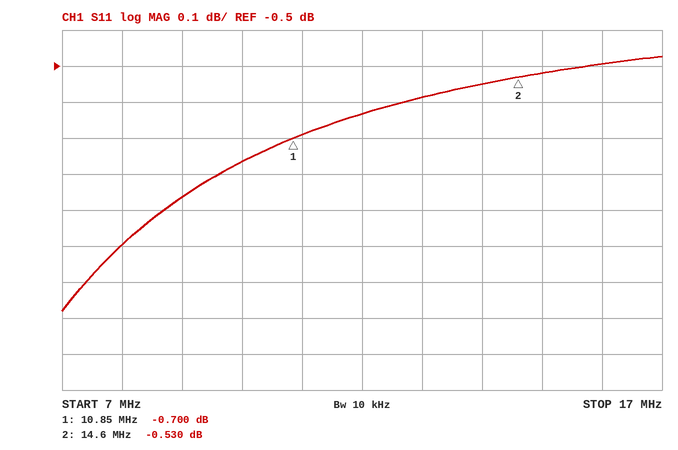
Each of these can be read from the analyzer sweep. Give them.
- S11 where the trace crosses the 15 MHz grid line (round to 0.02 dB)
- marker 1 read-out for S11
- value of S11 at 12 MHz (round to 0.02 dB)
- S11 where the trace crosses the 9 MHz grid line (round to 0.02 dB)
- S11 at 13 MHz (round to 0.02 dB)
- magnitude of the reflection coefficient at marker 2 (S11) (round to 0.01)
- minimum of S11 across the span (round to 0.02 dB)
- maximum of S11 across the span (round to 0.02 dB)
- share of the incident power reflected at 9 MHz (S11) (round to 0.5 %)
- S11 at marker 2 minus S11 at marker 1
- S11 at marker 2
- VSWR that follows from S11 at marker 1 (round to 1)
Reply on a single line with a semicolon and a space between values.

-0.52 dB; -0.700 dB; -0.64 dB; -0.86 dB; -0.58 dB; 0.94; -1.18 dB; -0.48 dB; 82.0 %; 0.170 dB; -0.530 dB; 25
